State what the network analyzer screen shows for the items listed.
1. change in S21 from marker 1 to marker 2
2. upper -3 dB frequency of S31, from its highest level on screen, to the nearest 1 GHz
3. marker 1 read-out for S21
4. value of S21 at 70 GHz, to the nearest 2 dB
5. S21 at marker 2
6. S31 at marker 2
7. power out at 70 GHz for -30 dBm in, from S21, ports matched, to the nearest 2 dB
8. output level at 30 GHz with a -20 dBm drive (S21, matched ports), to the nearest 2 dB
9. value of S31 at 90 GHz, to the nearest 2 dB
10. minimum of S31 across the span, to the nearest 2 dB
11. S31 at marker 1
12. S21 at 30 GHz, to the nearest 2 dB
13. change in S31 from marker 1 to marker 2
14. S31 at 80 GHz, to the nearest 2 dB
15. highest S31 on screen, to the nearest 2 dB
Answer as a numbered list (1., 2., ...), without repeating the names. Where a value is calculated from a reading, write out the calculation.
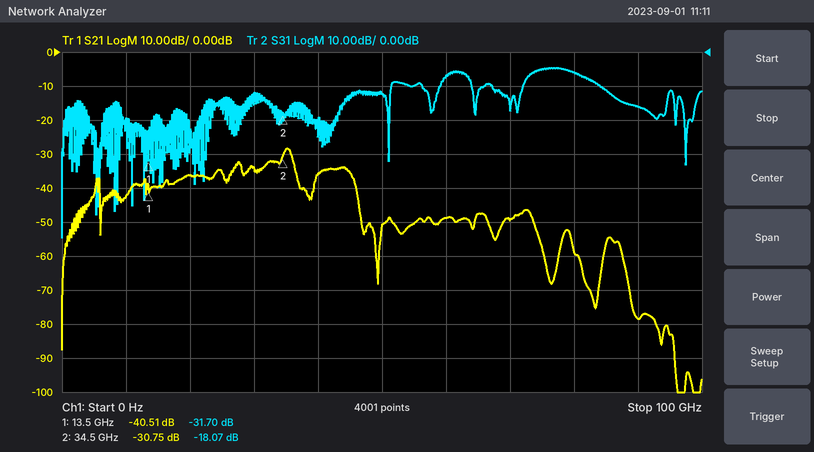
1. -30.75 − (-40.51) = 9.76 dB
2. 82 GHz
3. -40.51 dB
4. -50 dB
5. -30.75 dB
6. -18.07 dB
7. -30 dBm + (-50 dB) = -80 dBm
8. -20 dBm + (-34 dB) = -54 dBm
9. -16 dB
10. -54 dB
11. -31.70 dB
12. -34 dB
13. -18.07 − (-31.7) = 13.63 dB
14. -6 dB
15. -4 dB
